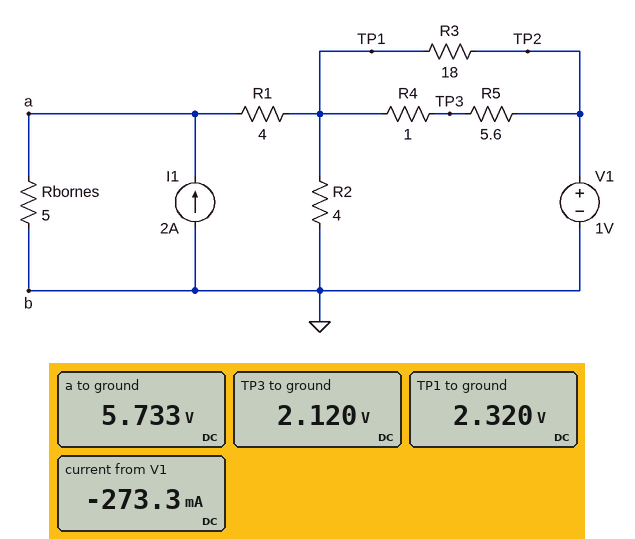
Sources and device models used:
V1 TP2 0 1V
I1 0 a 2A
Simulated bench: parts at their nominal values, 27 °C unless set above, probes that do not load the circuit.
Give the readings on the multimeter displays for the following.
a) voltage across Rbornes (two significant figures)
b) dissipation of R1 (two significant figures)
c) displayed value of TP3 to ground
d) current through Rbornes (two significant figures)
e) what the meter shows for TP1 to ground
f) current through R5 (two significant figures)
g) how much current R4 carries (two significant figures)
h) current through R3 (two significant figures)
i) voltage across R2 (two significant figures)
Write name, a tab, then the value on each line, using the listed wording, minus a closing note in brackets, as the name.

voltage across Rbornes	5.7 V
dissipation of R1	2.9 W
displayed value of TP3 to ground	2.120 V
current through Rbornes	1.1 A
what the meter shows for TP1 to ground	2.320 V
current through R5	200 mA
how much current R4 carries	200 mA
current through R3	73 mA
voltage across R2	2.3 V
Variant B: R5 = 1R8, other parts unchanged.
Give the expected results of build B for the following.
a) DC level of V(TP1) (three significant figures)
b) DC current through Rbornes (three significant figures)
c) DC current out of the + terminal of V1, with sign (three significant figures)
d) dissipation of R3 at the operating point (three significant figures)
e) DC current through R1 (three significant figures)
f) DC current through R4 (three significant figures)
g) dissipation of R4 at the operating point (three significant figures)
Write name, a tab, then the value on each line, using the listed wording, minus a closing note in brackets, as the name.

DC level of V(TP1)	1.97 V
DC current through Rbornes	1.11 A
DC current out of the + terminal of V1, with sign	-400 mA
dissipation of R3 at the operating point	52.2 mW
DC current through R1	892 mA
DC current through R4	346 mA
dissipation of R4 at the operating point	120 mW
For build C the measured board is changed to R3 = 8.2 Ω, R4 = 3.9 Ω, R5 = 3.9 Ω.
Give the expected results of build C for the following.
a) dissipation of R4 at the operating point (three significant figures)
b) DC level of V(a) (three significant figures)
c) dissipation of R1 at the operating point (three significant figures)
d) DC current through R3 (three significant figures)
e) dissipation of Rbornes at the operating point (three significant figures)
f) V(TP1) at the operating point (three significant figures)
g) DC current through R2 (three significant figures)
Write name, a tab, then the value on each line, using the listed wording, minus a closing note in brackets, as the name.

dissipation of R4 at the operating point	96.5 mW
DC level of V(a)	5.68 V
dissipation of R1 at the operating point	2.98 W
DC current through R3	150 mA
dissipation of Rbornes at the operating point	6.46 W
V(TP1) at the operating point	2.23 V
DC current through R2	557 mA
